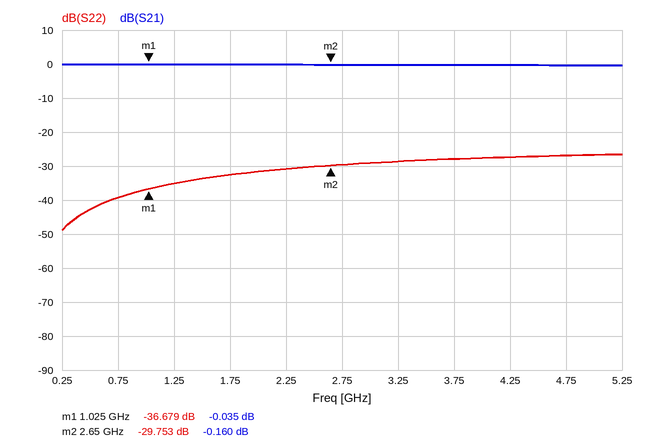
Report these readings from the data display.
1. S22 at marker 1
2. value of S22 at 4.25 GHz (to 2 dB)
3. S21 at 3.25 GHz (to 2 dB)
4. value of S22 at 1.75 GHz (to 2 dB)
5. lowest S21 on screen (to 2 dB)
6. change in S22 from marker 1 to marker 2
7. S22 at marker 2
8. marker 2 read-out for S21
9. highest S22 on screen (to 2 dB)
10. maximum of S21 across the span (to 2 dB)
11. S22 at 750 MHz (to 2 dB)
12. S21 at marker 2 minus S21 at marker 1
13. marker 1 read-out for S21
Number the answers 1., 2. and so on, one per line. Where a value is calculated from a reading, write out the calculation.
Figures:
1. -36.679 dB
2. -28 dB
3. 0 dB
4. -32 dB
5. 0 dB
6. -29.753 − (-36.679) = 6.926 dB
7. -29.753 dB
8. -0.160 dB
9. -26 dB
10. 0 dB
11. -40 dB
12. -0.16 − (-0.035) = -0.125 dB
13. -0.035 dB
